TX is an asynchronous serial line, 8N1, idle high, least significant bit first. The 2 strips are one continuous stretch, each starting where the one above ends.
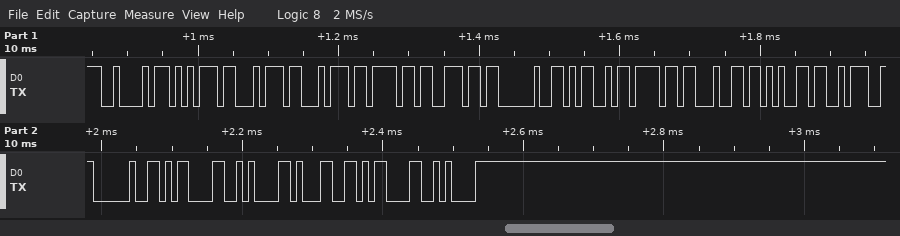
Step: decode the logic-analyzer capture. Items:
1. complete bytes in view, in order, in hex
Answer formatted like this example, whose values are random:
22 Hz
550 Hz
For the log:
0x42 0x75 0x74 0x74 0x6F 0x6E 0x20 0x4D 0x6F 0x64 0x65 0x3A 0x20 0x0D 0x0A 0x31 0x0D 0x0A
